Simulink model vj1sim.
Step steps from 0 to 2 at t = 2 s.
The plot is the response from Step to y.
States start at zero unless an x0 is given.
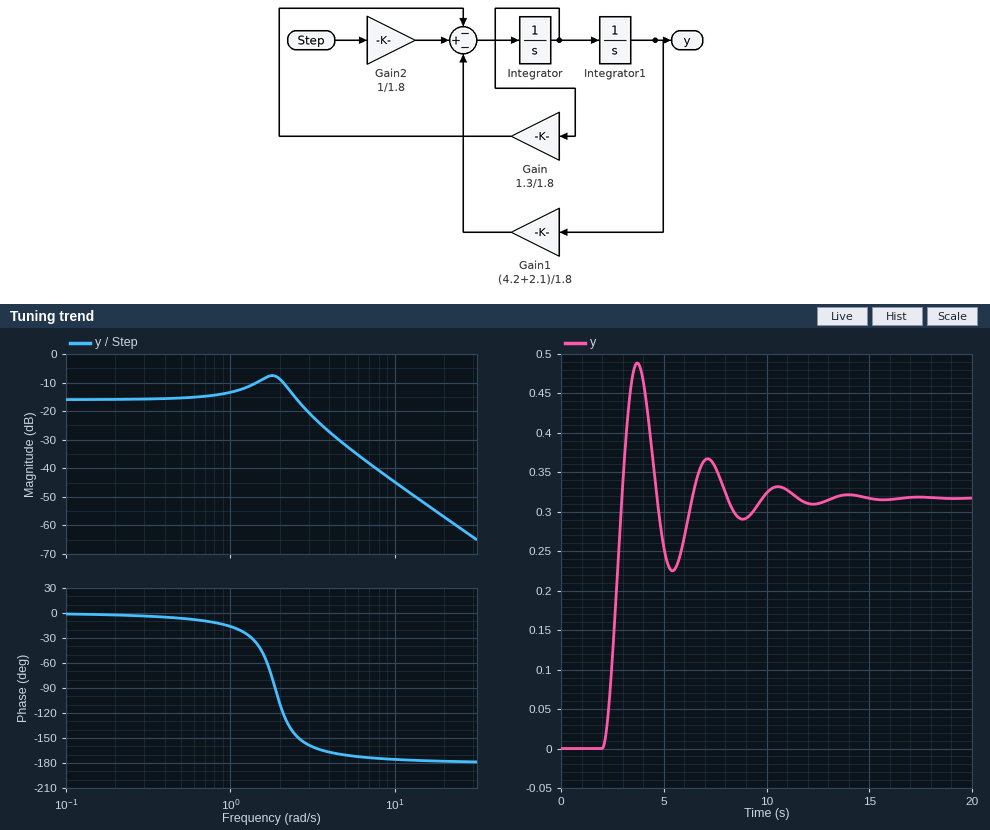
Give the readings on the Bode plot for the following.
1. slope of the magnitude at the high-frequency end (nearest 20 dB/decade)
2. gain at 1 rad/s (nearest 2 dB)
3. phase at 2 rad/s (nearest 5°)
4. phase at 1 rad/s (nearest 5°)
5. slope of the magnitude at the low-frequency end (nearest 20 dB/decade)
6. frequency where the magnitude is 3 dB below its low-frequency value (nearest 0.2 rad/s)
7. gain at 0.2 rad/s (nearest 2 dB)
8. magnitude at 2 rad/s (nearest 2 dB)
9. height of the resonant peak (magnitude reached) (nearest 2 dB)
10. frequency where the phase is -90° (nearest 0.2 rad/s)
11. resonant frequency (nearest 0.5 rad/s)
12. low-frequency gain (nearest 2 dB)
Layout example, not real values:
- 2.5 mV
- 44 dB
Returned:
- -40 dB/decade
- -14 dB
- -110°
- -15°
- 0 dB/decade
- 2.8 rad/s
- -16 dB
- -8 dB
- -8 dB
- 1.8 rad/s
- 2.0 rad/s
- -16 dB
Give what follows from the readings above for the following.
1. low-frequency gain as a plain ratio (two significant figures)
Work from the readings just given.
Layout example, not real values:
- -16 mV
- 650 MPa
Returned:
- 0.16
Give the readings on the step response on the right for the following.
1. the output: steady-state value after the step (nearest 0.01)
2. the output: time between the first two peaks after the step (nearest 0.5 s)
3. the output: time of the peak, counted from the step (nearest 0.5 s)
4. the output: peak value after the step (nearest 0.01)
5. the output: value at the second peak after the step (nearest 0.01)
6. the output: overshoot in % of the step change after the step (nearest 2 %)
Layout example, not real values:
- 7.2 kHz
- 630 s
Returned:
- 0.32
- 3.5 s
- 1.5 s
- 0.49
- 0.37
- 54 %
